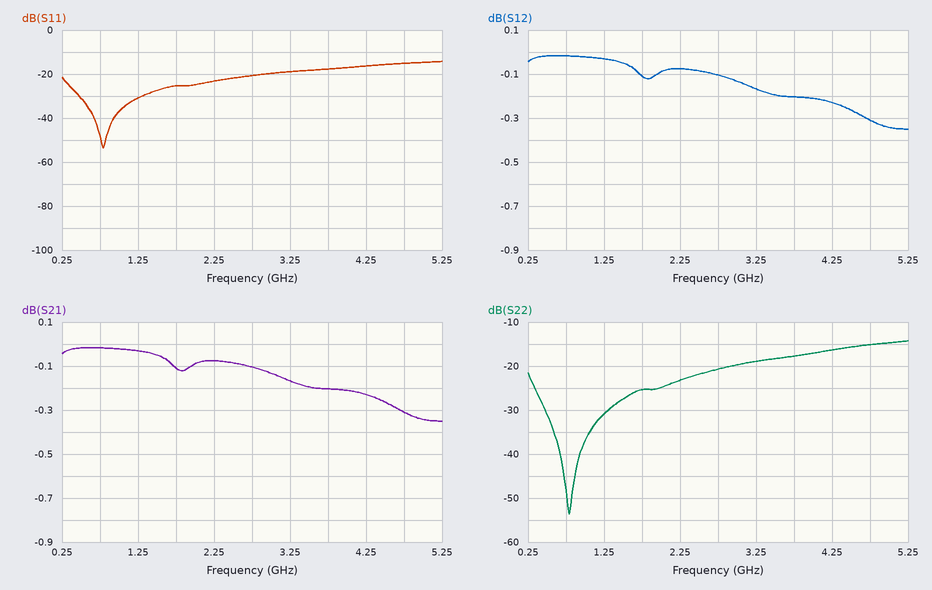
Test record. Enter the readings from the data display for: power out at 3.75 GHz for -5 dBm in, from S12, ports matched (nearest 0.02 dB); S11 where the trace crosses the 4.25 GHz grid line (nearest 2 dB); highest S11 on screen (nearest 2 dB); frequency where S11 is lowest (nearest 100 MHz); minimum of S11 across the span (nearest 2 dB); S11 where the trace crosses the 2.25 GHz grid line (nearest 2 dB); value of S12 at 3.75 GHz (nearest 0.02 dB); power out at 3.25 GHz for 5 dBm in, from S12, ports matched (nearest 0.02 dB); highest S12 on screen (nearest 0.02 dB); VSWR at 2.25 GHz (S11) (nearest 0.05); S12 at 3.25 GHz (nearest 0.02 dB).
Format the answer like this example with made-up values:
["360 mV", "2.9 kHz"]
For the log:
["-5.20 dBm", "-16 dB", "-14 dB", "800 MHz", "-54 dB", "-24 dB", "-0.20 dB", "4.84 dBm", "-0.02 dB", "1.15", "-0.16 dB"]
